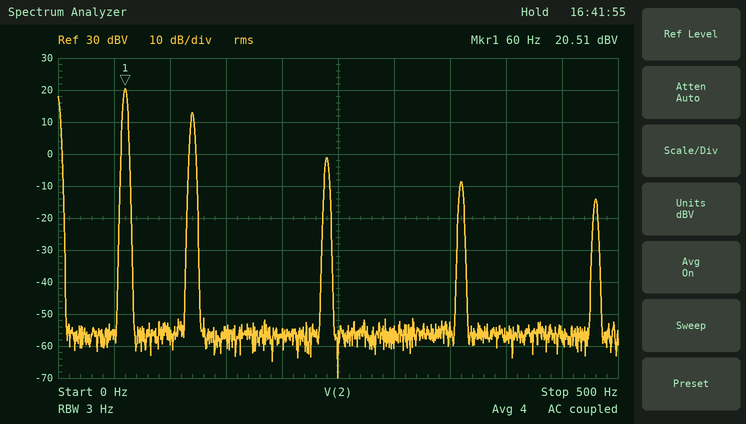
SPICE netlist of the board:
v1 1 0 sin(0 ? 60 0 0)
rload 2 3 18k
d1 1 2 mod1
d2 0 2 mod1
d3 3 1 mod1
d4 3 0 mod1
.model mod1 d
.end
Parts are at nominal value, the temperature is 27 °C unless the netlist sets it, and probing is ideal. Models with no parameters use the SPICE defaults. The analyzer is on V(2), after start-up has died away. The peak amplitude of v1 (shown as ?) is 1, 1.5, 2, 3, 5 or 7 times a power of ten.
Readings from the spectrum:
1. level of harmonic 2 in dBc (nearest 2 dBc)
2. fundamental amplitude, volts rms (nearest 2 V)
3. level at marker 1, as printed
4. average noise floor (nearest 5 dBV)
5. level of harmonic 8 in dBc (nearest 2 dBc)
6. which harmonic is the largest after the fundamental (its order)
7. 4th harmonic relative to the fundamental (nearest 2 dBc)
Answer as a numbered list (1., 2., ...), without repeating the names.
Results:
1. -8 dBc
2. 10 V
3. 20.51 dBV
4. -55 dBV
5. -34 dBc
6. 2
7. -22 dBc
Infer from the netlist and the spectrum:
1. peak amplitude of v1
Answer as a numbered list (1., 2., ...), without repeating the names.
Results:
1. 30 V
